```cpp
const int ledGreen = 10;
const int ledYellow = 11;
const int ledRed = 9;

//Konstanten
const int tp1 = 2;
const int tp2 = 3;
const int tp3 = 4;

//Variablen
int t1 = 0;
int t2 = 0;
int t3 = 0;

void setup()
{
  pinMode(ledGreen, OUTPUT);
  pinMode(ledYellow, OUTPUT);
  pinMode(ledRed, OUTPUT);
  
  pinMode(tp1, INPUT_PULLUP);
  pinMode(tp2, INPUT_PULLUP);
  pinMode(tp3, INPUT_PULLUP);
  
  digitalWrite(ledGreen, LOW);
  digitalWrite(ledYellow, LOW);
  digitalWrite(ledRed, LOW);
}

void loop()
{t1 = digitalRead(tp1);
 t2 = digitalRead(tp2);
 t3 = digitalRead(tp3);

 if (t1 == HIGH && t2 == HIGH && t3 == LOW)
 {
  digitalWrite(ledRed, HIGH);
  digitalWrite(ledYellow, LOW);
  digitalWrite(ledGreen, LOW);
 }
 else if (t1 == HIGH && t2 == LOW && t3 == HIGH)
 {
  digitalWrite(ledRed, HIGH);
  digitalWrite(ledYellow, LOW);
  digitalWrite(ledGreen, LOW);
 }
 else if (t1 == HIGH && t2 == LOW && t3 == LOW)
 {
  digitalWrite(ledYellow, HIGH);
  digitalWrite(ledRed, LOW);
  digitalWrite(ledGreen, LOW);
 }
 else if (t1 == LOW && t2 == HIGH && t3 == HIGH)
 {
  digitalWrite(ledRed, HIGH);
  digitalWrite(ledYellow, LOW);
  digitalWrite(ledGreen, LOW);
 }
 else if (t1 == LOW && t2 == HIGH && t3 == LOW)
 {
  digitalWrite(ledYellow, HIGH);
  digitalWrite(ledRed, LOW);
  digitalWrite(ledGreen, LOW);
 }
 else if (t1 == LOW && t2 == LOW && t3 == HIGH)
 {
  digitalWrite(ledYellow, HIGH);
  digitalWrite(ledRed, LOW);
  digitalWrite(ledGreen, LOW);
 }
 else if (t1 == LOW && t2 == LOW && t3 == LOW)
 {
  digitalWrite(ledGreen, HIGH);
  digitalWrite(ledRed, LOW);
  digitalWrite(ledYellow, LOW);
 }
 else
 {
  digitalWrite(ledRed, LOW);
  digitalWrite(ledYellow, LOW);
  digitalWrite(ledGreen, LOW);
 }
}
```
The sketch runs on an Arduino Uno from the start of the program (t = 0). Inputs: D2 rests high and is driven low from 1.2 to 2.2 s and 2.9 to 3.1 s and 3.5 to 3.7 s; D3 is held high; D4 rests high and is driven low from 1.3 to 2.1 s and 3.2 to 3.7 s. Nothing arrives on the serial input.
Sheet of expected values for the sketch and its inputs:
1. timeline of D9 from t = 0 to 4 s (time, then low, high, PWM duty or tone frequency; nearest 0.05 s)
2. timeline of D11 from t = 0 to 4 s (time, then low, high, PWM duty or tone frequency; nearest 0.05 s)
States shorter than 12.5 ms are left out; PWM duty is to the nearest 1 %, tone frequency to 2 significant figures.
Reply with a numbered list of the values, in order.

1. 0 s low; 1.2 s high; 1.3 s low; 2.1 s high; 2.2 s low; 2.9 s high; 3.1 s low; 3.2 s high; 3.5 s low
2. 0 s low; 1.3 s high; 2.1 s low; 3.5 s high; 3.7 s low
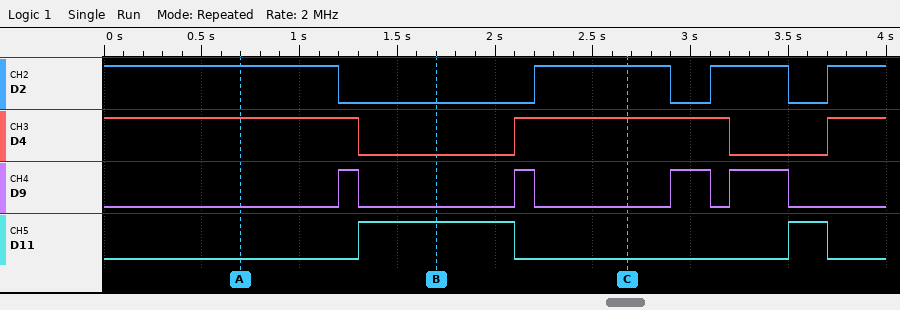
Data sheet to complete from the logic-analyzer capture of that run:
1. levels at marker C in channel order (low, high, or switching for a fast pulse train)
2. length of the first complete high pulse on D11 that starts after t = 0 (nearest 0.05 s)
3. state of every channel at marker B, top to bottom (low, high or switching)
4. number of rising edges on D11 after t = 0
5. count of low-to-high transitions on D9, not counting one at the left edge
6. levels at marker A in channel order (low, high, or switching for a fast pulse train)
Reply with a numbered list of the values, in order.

1. D2 high, D4 high, D9 low, D11 low
2. 0.80 s
3. D2 low, D4 low, D9 low, D11 high
4. 2
5. 4
6. D2 high, D4 high, D9 low, D11 low
